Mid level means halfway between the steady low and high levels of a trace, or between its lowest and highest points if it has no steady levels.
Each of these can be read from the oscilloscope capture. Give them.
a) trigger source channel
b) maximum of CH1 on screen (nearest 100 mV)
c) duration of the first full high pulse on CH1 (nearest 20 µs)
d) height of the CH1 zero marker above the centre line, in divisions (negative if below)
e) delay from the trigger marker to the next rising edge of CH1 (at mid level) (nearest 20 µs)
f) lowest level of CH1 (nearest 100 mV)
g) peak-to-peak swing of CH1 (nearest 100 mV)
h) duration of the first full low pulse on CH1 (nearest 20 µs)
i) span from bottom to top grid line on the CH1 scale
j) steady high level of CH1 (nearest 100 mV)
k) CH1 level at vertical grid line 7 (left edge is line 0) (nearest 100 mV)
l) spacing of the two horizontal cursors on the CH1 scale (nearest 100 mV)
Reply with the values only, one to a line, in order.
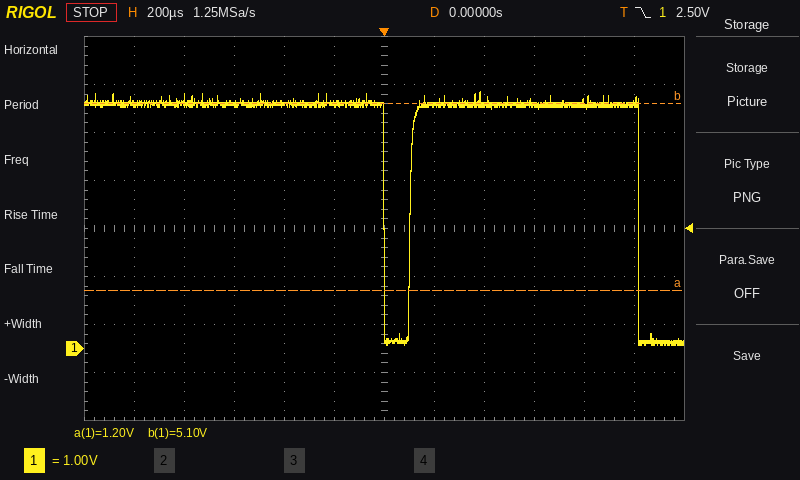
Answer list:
CH1
5.4 V
920 µs
-2.5 div
100 µs
100 mV
5.3 V
100 µs
8 V
5.1 V
5.1 V
3.9 V
